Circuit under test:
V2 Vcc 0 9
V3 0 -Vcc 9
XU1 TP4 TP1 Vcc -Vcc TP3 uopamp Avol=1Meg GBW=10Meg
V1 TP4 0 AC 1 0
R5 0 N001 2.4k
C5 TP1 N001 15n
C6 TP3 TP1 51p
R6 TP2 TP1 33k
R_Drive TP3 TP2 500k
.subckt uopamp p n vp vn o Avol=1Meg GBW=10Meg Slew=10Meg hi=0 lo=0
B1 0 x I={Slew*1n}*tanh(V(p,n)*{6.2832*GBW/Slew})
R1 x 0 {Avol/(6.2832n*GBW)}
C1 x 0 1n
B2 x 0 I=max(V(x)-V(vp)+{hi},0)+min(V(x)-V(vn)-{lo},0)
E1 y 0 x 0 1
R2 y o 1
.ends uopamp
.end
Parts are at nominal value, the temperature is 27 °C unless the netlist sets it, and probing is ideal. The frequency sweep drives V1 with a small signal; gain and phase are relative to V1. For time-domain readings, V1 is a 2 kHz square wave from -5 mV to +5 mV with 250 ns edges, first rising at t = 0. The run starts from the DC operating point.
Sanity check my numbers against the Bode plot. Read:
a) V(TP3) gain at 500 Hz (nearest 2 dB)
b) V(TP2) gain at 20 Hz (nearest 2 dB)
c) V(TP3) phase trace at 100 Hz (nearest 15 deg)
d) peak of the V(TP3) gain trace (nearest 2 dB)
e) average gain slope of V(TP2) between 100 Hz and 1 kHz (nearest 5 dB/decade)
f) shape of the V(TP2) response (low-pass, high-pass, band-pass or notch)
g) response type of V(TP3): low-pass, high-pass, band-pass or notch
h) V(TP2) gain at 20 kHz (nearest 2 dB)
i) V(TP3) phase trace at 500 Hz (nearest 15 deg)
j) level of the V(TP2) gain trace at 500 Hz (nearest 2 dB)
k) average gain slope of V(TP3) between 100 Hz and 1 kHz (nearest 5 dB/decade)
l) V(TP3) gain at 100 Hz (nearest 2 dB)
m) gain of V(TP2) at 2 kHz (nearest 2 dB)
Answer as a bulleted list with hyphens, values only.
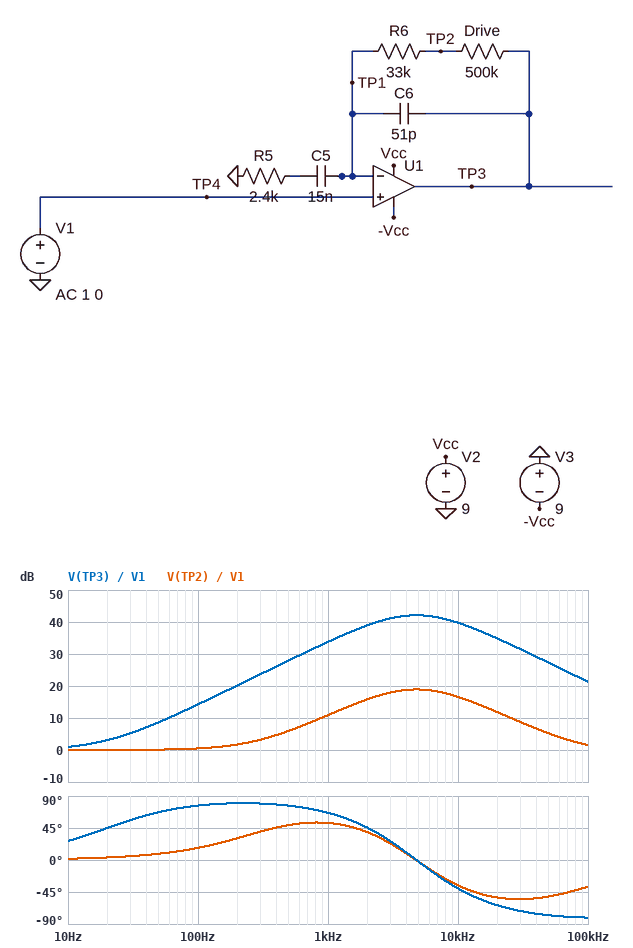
- 28 dB
- 0 dB
- 75 deg
- 42 dB
- 10 dB/decade
- band-pass
- band-pass
- 12 dB
- 75 deg
- 6 dB
- 20 dB/decade
- 14 dB
- 16 dB
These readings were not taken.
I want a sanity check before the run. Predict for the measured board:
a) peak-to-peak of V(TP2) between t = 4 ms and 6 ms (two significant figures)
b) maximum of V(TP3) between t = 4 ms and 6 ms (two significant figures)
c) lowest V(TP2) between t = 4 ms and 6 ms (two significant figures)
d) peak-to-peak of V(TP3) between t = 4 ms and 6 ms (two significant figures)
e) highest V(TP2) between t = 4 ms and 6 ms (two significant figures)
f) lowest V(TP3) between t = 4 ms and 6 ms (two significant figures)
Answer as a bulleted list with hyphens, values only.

- 120 mV
- 920 mV
- -62 mV
- 1.8 V
- 62 mV
- -920 mV
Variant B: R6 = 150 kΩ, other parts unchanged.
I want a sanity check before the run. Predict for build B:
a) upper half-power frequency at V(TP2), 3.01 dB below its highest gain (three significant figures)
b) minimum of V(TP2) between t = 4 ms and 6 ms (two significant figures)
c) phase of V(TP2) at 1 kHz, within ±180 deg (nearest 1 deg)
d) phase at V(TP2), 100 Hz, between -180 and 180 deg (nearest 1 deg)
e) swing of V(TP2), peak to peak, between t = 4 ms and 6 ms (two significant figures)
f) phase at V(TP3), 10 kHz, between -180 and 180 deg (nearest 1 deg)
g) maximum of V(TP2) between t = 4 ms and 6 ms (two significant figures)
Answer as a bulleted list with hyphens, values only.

- 10.0 kHz
- -240 mV
- 62 deg
- 53 deg
- 480 mV
- -45 deg
- 240 mV
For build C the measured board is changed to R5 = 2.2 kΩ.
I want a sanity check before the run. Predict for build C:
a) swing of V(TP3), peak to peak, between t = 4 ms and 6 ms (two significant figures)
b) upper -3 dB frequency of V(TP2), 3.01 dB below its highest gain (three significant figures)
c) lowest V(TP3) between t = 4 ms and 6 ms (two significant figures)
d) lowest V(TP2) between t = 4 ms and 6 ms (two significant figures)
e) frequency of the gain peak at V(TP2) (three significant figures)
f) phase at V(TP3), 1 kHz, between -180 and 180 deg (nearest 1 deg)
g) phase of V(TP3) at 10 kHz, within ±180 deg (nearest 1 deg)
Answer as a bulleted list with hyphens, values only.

- 1.9 V
- 11.6 kHz
- -960 mV
- -64 mV
- 4.97 kHz
- 67 deg
- -39 deg
